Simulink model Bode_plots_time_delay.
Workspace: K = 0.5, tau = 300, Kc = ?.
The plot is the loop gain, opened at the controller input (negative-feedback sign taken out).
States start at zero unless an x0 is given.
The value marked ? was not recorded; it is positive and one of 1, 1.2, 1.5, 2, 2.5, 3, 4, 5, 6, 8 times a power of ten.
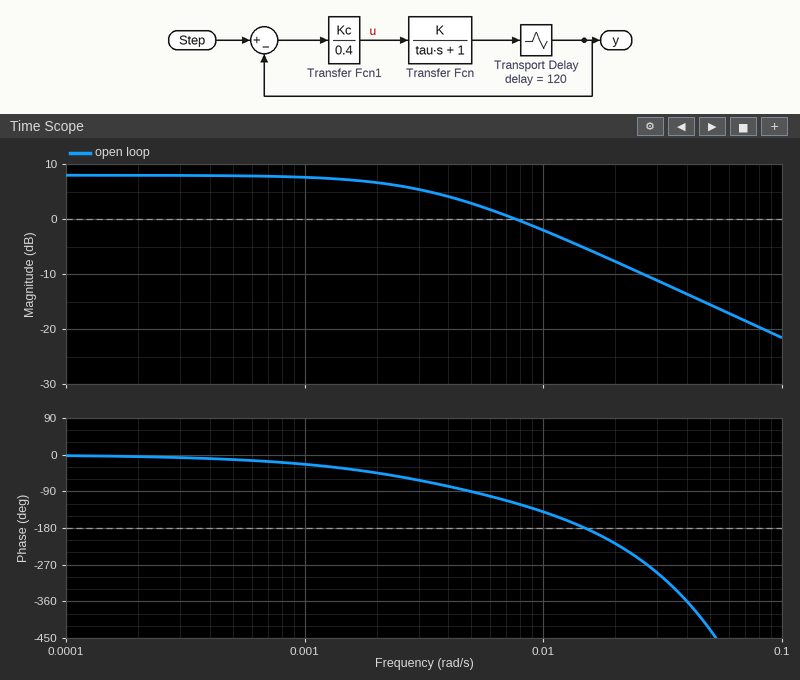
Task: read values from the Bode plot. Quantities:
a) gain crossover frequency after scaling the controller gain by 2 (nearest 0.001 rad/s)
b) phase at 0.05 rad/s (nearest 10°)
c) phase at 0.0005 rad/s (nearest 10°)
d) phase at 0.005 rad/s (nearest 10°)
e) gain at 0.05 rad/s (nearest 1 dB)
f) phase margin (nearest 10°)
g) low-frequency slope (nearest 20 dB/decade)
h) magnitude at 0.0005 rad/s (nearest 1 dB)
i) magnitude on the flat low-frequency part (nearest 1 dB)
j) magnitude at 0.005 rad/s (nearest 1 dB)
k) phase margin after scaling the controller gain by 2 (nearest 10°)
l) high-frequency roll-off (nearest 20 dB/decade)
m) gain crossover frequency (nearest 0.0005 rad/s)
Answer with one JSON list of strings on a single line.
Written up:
["0.016 rad/s", "-430°", "-10°", "-90°", "-16 dB", "60°", "0 dB/decade", "8 dB", "8 dB", "3 dB", "-10°", "-20 dB/decade", "0.0075 rad/s"]
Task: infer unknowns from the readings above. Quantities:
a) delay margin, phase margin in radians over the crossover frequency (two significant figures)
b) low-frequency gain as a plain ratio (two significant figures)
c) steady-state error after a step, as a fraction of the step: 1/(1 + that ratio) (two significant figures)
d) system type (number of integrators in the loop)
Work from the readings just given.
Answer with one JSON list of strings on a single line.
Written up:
["140 s", "2.5", "0.29", "0"]
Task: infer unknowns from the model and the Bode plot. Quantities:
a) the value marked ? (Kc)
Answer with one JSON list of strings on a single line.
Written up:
["2"]
